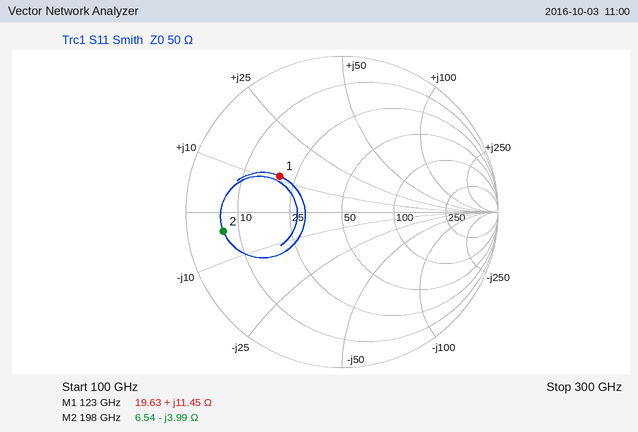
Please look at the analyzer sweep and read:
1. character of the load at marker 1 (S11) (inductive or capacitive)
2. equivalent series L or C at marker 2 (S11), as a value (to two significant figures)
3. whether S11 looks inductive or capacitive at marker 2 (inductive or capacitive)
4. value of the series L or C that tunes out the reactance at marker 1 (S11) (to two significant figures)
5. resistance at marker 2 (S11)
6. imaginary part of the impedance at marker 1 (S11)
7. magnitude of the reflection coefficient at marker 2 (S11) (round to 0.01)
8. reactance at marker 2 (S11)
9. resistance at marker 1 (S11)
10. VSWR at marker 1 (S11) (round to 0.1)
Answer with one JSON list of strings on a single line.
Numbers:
["inductive", "200 fF", "capacitive", "110 fF", "6.54 Ω", "+11.45 Ω", "0.77", "-3.99 Ω", "19.63 Ω", "2.7"]
